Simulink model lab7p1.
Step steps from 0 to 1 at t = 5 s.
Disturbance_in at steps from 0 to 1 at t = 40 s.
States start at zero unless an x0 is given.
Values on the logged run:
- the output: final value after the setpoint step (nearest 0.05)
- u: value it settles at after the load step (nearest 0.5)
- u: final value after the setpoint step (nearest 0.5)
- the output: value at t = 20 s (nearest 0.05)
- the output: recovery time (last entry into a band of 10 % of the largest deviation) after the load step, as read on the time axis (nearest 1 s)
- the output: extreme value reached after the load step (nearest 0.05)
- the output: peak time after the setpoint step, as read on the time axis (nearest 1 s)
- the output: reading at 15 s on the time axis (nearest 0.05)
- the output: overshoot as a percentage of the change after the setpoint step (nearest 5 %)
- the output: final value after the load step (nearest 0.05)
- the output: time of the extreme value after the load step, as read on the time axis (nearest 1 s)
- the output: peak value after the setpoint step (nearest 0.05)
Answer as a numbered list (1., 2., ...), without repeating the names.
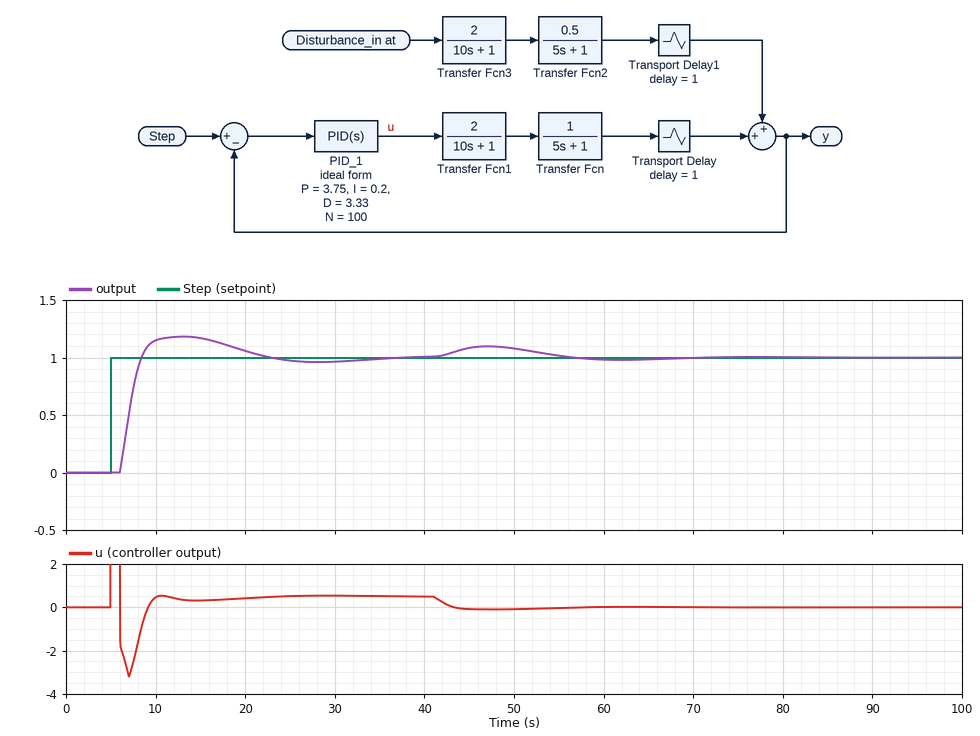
1. 1.00
2. 0.0
3. 0.5
4. 1.05
5. 68 s
6. 1.10
7. 13 s
8. 1.15
9. 20 %
10. 1.00
11. 47 s
12. 1.20
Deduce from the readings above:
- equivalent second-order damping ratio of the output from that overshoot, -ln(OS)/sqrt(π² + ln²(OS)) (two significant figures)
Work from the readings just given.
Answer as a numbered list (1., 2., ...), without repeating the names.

1. 0.46
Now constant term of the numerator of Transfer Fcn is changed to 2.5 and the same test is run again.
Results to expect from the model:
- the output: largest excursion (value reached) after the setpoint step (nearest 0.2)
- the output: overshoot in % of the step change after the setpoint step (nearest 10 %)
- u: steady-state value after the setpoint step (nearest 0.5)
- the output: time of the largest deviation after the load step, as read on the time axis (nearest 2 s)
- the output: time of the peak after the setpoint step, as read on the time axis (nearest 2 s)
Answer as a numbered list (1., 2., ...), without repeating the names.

1. 1.8
2. 80 %
3. 0.0
4. 44 s
5. 8 s
